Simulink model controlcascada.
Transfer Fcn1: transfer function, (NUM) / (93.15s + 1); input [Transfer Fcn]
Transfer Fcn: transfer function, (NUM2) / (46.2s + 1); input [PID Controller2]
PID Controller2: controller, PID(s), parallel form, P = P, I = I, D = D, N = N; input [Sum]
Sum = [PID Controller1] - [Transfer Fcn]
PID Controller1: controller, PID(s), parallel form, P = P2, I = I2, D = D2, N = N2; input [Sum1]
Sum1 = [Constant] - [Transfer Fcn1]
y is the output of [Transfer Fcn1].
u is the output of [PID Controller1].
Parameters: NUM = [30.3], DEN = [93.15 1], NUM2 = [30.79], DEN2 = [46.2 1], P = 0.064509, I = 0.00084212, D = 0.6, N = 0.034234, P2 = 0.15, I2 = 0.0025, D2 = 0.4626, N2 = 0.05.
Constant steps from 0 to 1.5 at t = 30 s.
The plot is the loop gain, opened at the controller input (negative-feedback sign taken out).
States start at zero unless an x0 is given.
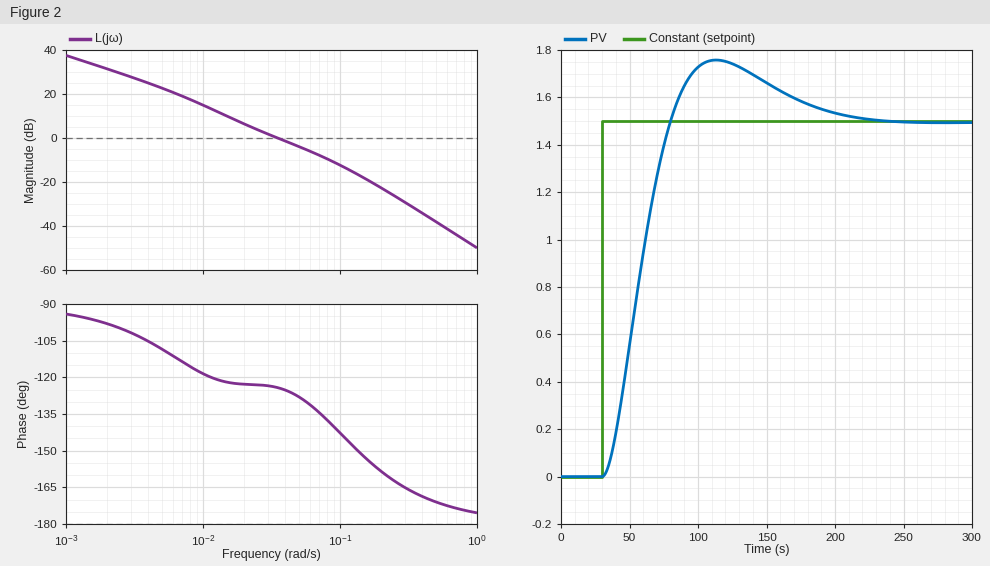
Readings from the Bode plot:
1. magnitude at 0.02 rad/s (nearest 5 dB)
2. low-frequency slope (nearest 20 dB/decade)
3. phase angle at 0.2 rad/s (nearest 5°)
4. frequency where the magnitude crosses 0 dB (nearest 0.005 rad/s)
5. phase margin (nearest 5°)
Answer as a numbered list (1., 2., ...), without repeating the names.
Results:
1. 5 dB
2. -20 dB/decade
3. -160°
4. 0.035 rad/s
5. 55°
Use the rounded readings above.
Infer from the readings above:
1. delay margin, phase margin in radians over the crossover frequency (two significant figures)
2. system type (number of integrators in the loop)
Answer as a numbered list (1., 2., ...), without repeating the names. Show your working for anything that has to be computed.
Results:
1. 55 × π / 180 / 0.035 = 27 s
2. 1
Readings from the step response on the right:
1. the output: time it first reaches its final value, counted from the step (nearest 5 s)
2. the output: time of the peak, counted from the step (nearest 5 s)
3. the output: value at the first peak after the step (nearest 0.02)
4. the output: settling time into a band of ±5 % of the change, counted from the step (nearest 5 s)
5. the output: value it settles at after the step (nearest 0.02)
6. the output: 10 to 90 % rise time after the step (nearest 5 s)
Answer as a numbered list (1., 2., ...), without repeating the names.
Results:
1. 50 s
2. 85 s
3. 1.76
4. 150 s
5. 1.50
6. 35 s
